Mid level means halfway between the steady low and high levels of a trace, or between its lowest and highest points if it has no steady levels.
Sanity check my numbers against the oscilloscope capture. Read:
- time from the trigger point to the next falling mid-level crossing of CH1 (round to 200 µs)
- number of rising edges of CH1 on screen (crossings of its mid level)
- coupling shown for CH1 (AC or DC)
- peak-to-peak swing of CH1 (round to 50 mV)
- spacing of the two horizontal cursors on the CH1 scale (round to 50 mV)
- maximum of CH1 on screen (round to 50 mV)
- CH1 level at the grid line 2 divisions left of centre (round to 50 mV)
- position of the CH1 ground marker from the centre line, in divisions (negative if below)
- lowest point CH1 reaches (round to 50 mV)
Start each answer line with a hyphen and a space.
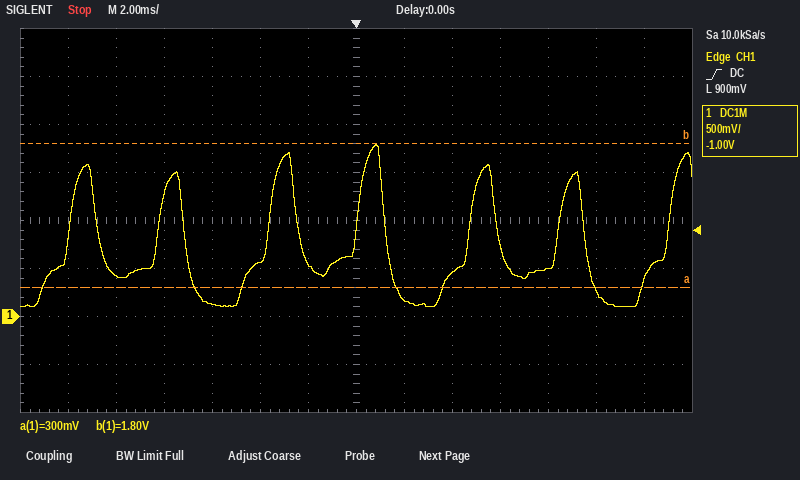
- 1.2 ms
- 7
- DC
- 1.70 V
- 1.50 V
- 1.80 V
- 550 mV
- -2.0 div
- 100 mV
